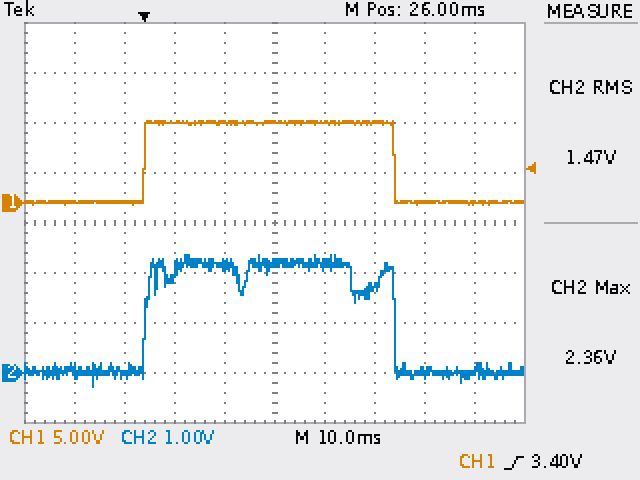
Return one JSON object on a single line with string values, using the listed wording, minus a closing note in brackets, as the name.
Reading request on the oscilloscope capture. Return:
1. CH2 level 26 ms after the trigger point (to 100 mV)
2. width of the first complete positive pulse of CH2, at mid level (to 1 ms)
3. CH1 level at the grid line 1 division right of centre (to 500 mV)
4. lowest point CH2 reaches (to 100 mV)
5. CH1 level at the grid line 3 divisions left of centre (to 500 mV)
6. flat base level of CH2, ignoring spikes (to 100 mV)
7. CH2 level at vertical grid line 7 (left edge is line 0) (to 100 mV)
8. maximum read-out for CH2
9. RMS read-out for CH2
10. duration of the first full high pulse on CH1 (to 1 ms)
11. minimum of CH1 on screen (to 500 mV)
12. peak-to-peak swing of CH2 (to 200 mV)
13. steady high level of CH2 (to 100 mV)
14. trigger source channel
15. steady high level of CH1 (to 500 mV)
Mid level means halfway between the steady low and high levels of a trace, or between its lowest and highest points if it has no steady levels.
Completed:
{"CH2 level 26 ms after the trigger point": "2.2 V", "width of the first complete positive pulse of CH2, at mid level": "50 ms", "CH1 level at the grid line 1 division right of centre": "8.0 V", "lowest point CH2 reaches": "-300 mV", "CH1 level at the grid line 3 divisions left of centre": "0.0 V", "flat base level of CH2, ignoring spikes": "0.0 V", "CH2 level at vertical grid line 7 (left edge is line 0)": "1.7 V", "maximum read-out for CH2": "2.36 V", "RMS read-out for CH2": "1.47 V", "duration of the first full high pulse on CH1": "50 ms", "minimum of CH1 on screen": "0.0 V", "peak-to-peak swing of CH2": "2.6 V", "steady high level of CH2": "2.2 V", "trigger source channel": "CH1", "steady high level of CH1": "8.0 V"}
